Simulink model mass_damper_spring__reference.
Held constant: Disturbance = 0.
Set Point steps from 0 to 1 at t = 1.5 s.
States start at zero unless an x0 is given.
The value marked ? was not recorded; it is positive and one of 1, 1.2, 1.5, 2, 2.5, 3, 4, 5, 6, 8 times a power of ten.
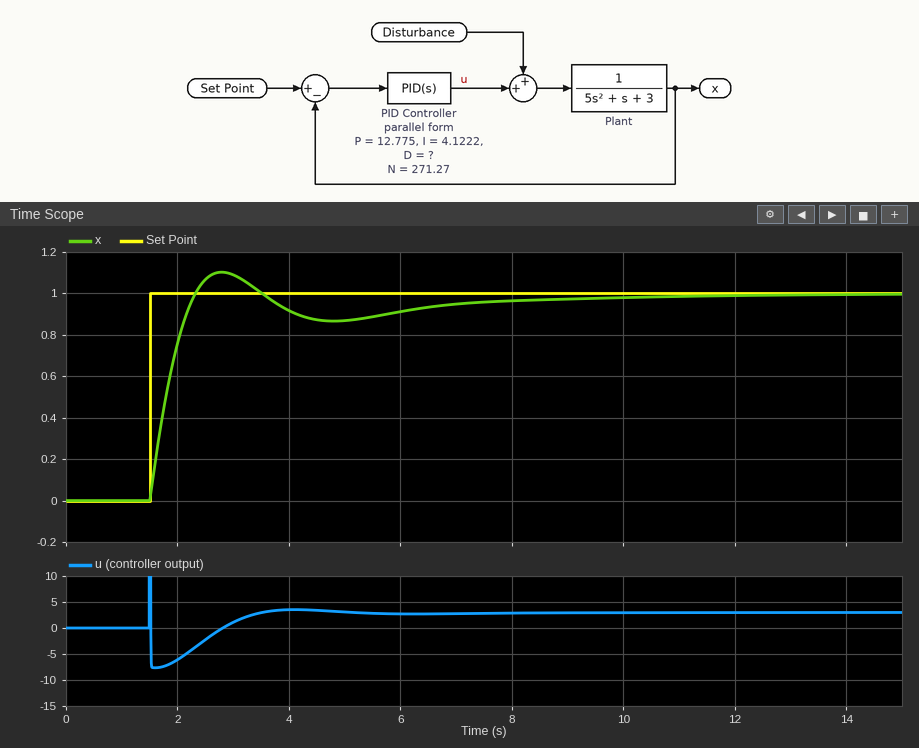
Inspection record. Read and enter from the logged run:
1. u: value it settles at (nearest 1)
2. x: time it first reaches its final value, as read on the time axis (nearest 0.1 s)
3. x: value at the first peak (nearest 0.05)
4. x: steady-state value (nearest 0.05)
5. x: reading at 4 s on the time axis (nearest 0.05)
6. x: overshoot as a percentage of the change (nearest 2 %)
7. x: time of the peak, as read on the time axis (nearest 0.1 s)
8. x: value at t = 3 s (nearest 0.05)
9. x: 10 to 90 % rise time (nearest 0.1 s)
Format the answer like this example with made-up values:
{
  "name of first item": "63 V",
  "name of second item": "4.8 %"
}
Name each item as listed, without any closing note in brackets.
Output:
{
  "u: value it settles at": "3",
  "x: time it first reaches its final value, as read on the time axis": "2.3 s",
  "x: value at the first peak": "1.10",
  "x: steady-state value": "1.00",
  "x: reading at 4 s on the time axis": "0.90",
  "x: overshoot as a percentage of the change": "10 %",
  "x: time of the peak, as read on the time axis": "2.8 s",
  "x: value at t = 3 s": "1.10",
  "x: 10 to 90 % rise time": "0.6 s"
}
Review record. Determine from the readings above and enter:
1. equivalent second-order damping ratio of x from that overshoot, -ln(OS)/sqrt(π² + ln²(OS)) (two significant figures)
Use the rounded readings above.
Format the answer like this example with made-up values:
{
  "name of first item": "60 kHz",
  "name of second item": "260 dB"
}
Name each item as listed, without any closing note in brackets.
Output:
{
  "equivalent second-order damping ratio of x from that overshoot, -ln(OS)/sqrt(π² + ln²(OS))": "0.59"
}
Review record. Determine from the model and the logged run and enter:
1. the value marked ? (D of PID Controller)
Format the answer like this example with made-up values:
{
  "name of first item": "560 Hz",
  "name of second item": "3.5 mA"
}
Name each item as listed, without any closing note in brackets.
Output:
{
  "the value marked ?": "10"
}
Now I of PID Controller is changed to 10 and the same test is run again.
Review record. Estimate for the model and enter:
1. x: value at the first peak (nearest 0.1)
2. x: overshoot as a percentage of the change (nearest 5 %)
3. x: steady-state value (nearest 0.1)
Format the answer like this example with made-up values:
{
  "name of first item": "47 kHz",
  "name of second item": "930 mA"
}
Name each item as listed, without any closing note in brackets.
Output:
{
  "x: value at the first peak": "1.2",
  "x: overshoot as a percentage of the change": "20 %",
  "x: steady-state value": "1.0"
}
